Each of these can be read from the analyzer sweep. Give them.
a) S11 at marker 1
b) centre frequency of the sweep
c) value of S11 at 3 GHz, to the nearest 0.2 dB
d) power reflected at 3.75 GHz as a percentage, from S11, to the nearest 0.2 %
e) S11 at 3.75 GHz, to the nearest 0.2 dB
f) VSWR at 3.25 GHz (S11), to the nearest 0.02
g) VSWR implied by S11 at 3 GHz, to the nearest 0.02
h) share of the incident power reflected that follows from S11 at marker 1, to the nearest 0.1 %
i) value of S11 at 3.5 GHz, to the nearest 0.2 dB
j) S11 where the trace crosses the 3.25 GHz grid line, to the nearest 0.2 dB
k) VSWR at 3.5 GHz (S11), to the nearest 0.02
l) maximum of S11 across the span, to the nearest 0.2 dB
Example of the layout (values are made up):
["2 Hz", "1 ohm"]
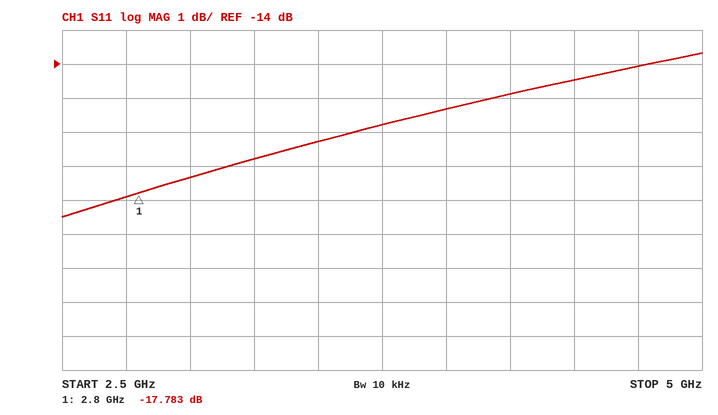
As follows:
["-17.783 dB", "3.75 GHz", "-17.4 dB", "2.6 %", "-15.8 dB", "1.34", "1.32", "1.7 %", "-16.2 dB", "-16.8 dB", "1.36", "-13.6 dB"]
